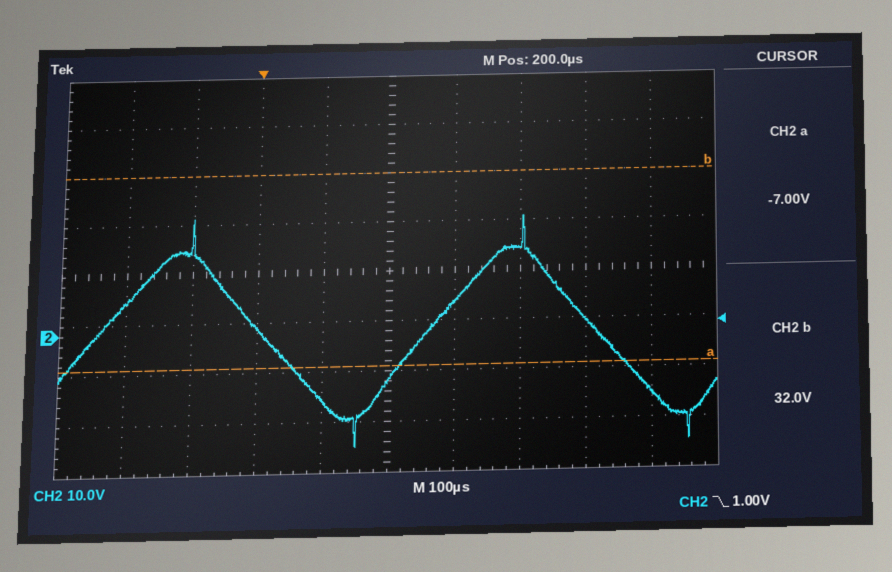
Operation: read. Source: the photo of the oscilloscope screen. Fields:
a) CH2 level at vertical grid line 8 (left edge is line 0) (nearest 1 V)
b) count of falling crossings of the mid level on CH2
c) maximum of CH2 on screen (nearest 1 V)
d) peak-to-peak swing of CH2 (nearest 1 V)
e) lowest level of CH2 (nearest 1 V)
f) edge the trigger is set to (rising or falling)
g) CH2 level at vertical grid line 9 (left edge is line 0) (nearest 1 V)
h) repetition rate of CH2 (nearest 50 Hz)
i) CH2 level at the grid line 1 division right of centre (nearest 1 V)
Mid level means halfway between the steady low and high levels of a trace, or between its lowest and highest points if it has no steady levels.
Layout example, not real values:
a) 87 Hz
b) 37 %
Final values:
a) 2 V
b) 2
c) 23 V
d) 46 V
e) -23 V
f) falling
g) -13 V
h) 2.00 kHz
i) 6 V
